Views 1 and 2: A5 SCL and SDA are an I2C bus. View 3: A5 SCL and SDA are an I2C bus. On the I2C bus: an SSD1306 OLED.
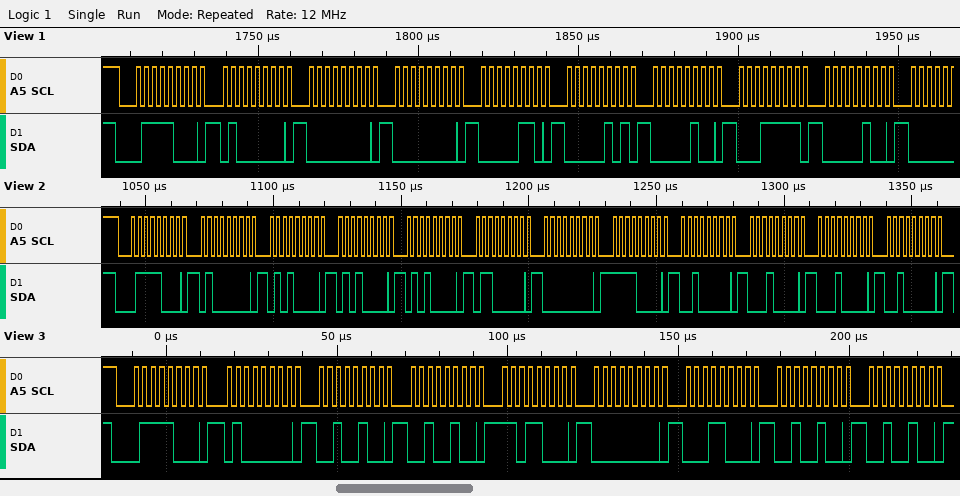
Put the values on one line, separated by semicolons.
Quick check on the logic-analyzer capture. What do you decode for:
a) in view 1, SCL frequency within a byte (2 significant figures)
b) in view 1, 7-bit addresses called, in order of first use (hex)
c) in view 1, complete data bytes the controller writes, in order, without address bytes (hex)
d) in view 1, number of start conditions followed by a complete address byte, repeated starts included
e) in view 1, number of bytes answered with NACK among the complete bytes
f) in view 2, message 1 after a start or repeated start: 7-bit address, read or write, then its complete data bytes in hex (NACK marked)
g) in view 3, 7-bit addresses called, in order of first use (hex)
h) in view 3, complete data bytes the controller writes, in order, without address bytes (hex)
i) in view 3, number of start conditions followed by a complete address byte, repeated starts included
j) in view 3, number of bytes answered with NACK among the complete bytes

400 kHz; 0x3C; 40 00 00 06 05 04 1F 04; 1; 0; 0x3C write: 40 50 50 50 60 00 F0 20 10 10 20; 0x3C; 40 24 24 D8 00 18 24 24; 1; 0
